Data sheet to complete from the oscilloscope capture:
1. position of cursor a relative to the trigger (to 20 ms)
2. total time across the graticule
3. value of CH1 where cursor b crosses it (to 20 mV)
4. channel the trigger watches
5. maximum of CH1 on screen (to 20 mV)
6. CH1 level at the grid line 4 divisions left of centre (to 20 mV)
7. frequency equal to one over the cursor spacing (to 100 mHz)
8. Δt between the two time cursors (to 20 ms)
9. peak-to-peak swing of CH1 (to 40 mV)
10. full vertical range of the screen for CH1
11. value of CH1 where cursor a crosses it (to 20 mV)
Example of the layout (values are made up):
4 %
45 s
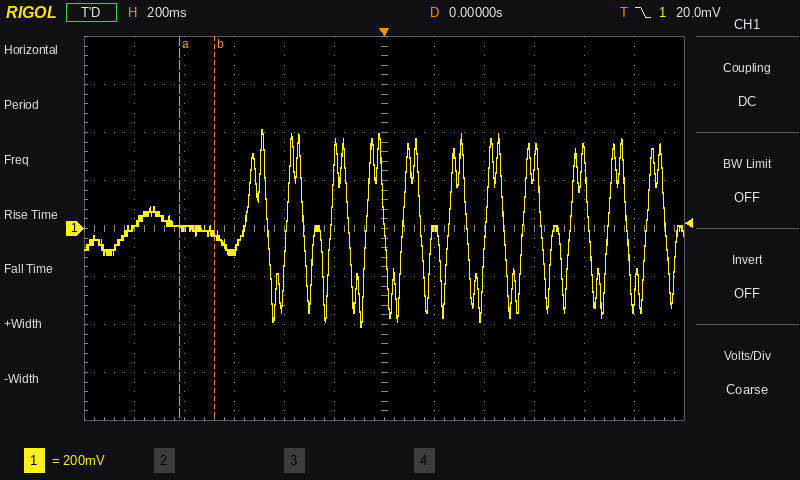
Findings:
-820 ms
2.4 s
-20 mV
CH1
420 mV
0 mV
7.1 Hz
140 ms
840 mV
1.6 V
0 mV
